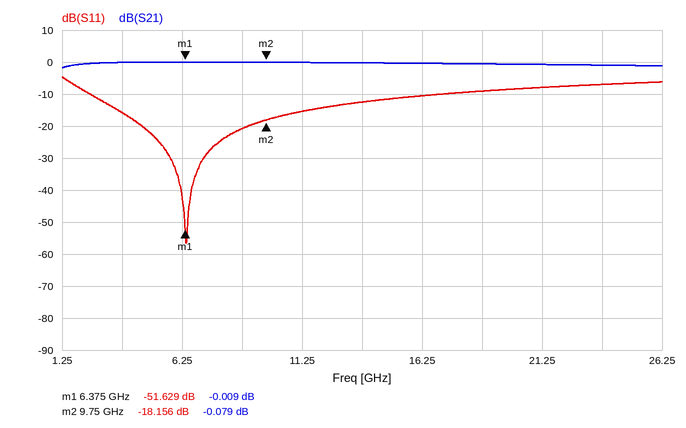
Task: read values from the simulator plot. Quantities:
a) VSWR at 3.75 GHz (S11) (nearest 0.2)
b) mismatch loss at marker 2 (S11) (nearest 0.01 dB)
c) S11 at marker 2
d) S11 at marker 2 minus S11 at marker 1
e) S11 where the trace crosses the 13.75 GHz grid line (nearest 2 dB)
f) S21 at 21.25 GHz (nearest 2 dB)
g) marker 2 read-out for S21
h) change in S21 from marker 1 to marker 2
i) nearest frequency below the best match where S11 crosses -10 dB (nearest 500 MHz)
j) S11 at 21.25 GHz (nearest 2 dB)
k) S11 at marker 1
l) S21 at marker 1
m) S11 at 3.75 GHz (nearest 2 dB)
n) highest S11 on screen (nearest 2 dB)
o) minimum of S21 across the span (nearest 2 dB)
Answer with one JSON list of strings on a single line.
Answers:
["1.4", "0.07 dB", "-18.156 dB", "33.473 dB", "-12 dB", "0 dB", "-0.079 dB", "-0.070 dB", "2.5 GHz", "-8 dB", "-51.629 dB", "-0.009 dB", "-16 dB", "-4 dB", "-2 dB"]
